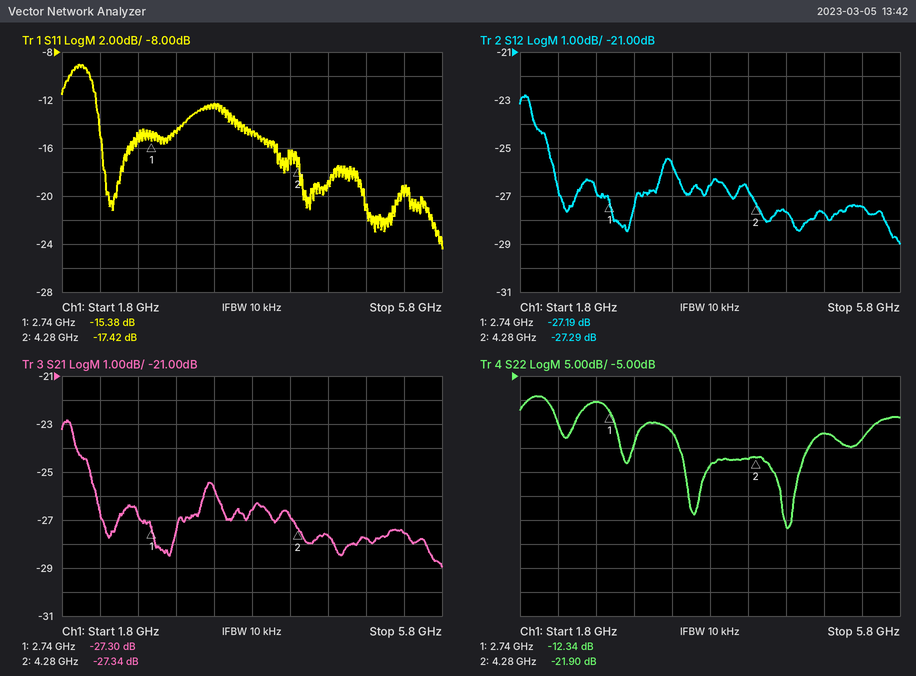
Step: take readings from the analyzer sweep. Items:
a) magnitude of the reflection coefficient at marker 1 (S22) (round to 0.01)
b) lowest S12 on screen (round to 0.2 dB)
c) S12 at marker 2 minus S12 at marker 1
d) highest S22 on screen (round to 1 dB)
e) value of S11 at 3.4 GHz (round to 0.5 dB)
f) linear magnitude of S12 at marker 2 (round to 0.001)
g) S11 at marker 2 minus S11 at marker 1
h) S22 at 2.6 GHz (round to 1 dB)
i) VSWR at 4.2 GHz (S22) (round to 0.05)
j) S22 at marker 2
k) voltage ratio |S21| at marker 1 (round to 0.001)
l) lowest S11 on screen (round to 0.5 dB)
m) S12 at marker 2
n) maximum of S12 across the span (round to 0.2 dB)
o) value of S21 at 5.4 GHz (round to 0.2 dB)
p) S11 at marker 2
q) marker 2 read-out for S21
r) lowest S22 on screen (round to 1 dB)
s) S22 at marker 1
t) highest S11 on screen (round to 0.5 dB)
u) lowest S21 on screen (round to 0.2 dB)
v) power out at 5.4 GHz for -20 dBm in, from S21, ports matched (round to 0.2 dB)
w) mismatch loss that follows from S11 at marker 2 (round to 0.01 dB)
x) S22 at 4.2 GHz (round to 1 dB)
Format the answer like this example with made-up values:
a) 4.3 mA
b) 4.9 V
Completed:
a) 0.24
b) -29.0 dB
c) -0.10 dB
d) -9 dB
e) -12.5 dB
f) 0.043
g) -2.04 dB
h) -10 dB
i) 1.15
j) -21.90 dB
k) 0.043
l) -24.5 dB
m) -27.29 dB
n) -22.8 dB
o) -27.6 dB
p) -17.42 dB
q) -27.34 dB
r) -37 dB
s) -12.34 dB
t) -9.0 dB
u) -29.0 dB
v) -47.6 dBm
w) 0.08 dB
x) -22 dB
